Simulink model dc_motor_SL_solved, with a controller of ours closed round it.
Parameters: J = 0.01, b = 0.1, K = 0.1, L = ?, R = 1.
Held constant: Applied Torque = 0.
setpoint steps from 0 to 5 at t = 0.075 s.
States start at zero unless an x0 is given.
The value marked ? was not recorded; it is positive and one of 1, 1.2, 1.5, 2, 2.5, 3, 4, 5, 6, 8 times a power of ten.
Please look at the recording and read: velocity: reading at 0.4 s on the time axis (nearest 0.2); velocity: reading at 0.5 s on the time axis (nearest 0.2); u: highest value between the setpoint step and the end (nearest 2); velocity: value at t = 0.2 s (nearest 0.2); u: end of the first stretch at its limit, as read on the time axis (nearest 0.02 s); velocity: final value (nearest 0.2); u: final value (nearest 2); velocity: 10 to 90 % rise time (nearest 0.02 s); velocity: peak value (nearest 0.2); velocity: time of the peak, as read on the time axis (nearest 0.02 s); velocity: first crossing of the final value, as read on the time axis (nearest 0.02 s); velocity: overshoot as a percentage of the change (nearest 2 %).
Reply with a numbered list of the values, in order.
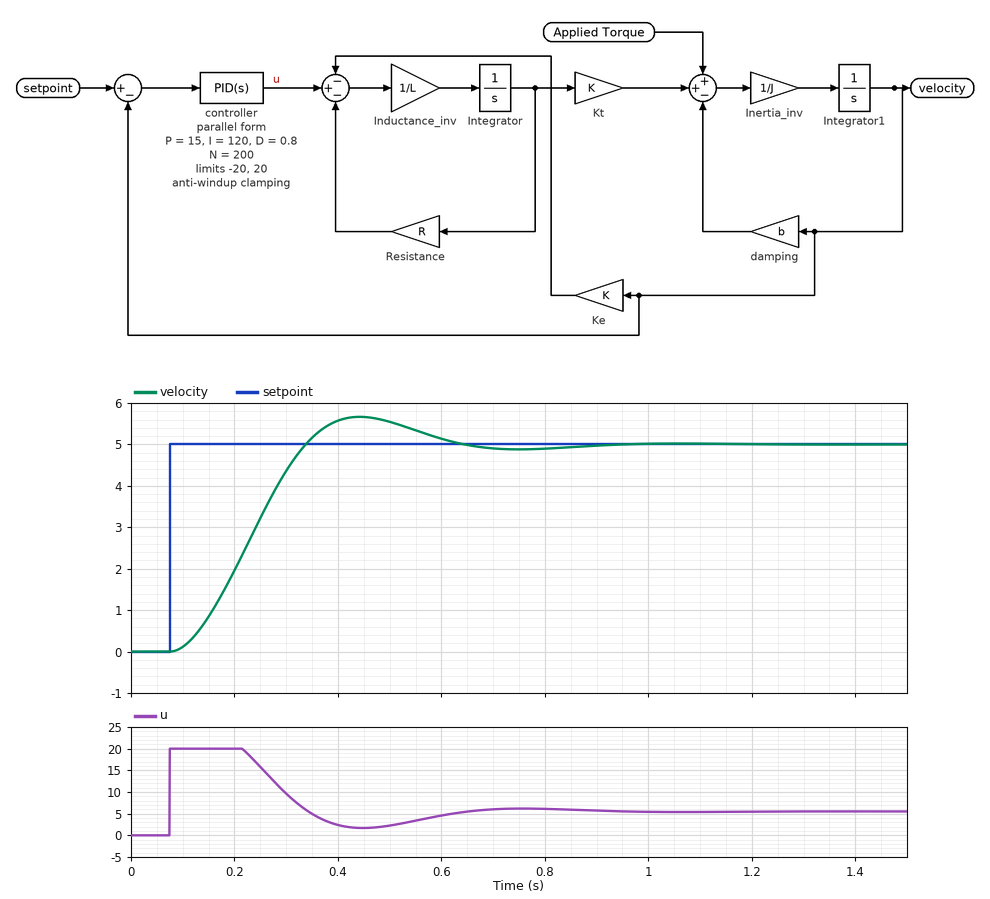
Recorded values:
1. 5.6
2. 5.6
3. 20
4. 2.0
5. 0.22 s
6. 5.0
7. 6
8. 0.18 s
9. 5.6
10. 0.44 s
11. 0.34 s
12. 14 %
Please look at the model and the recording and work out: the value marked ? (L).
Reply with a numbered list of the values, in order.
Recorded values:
1. 0.5
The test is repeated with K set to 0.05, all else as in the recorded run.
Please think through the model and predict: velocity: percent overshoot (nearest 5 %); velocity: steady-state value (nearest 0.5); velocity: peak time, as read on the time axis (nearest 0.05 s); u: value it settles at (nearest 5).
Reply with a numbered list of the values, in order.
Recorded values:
1. 10 %
2. 5.0
3. 0.70 s
4. 10
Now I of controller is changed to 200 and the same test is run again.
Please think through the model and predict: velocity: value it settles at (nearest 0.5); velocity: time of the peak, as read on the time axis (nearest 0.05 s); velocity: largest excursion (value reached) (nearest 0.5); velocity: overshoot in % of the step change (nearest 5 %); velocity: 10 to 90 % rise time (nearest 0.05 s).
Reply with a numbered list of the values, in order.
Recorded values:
1. 5.0
2. 0.40 s
3. 6.0
4. 20 %
5. 0.15 s
